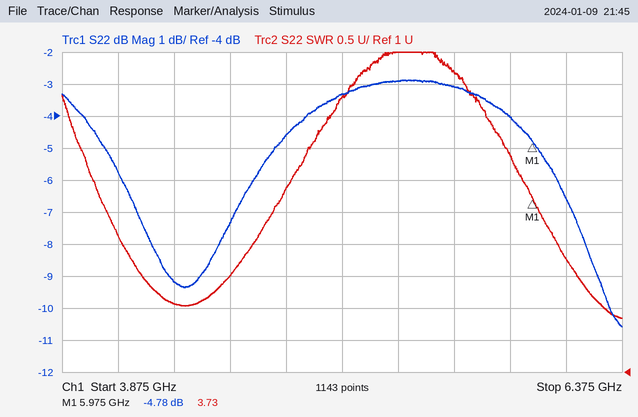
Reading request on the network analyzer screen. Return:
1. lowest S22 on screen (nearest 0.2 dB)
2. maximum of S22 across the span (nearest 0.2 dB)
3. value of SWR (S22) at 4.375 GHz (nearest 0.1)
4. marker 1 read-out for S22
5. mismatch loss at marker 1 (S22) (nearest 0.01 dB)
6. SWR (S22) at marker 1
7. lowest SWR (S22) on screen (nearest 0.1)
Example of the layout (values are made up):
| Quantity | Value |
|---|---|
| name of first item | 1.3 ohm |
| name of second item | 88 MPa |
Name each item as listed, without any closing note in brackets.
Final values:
| Quantity | Value |
|---|---|
| lowest S22 on screen | -10.6 dB |
| maximum of S22 across the span | -2.8 dB |
| value of SWR (S22) at 4.375 GHz | 2.1 |
| marker 1 read-out for S22 | -4.78 dB |
| mismatch loss at marker 1 (S22) | 1.76 dB |
| SWR (S22) at marker 1 | 3.73 |
| lowest SWR (S22) on screen | 1.8 |
